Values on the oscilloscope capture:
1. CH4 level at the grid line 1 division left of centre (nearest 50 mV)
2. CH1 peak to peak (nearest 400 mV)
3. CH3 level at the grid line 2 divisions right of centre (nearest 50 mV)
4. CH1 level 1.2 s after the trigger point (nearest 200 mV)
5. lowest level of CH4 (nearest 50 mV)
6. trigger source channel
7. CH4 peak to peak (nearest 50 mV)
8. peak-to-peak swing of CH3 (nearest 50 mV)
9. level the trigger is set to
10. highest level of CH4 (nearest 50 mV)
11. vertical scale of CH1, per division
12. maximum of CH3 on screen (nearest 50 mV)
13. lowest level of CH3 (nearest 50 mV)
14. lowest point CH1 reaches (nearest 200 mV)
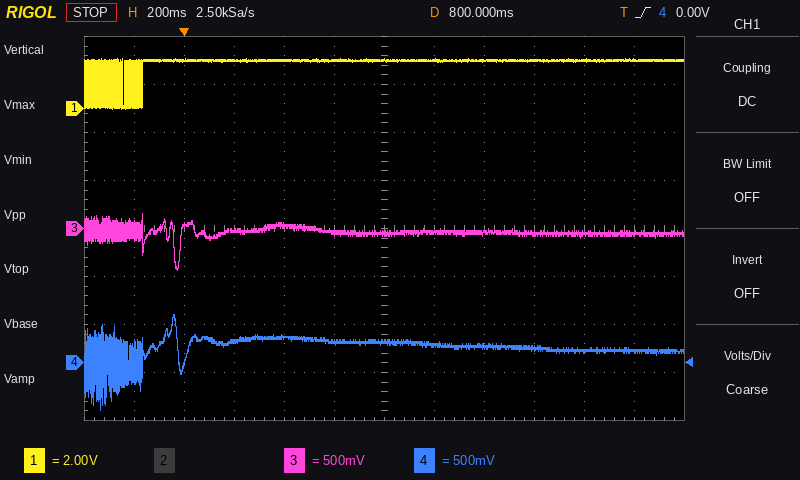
200 mV
2.0 V
-50 mV
2.0 V
-500 mV
CH4
1.00 V
600 mV
0.00 V
500 mV
2 V
150 mV
-450 mV
0.0 V
